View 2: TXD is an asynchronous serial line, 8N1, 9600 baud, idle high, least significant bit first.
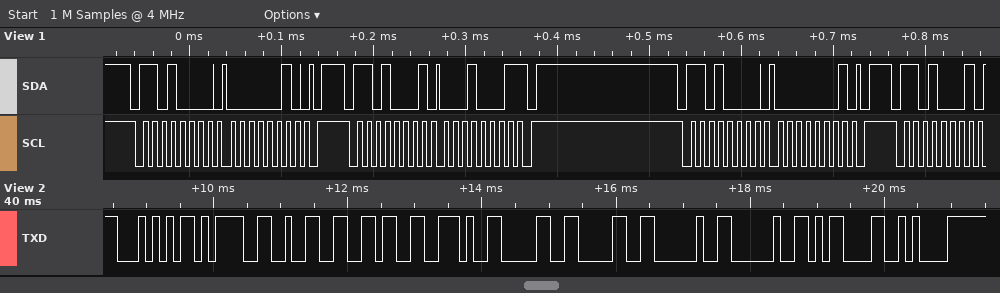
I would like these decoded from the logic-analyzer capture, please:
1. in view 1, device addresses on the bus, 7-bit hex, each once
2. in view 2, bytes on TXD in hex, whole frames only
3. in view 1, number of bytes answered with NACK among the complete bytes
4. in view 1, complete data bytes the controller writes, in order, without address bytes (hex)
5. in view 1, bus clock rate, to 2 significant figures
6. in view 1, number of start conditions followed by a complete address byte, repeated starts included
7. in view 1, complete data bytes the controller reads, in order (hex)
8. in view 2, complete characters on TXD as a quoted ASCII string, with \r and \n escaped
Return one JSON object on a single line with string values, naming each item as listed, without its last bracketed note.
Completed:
{"in view 1, device addresses on the bus, 7-bit hex, each once": "0x68", "in view 2, bytes on TXD in hex, whole frames only": "0x54 0x3D 0x32 0x36 0x2E 0x30 0x30 0x20 0x20 0x0D 0x0A", "in view 1, number of bytes answered with NACK among the complete bytes": "1", "in view 1, complete data bytes the controller writes, in order, without address bytes": "02 01", "in view 1, bus clock rate, to 2 significant figures": "100 kHz", "in view 1, number of start conditions followed by a complete address byte, repeated starts included": "4", "in view 1, complete data bytes the controller reads, in order": "11", "in view 2, complete characters on TXD as a quoted ASCII string, with \\r and \\n escaped": "\"T=26.00  \\r\\n\""}
